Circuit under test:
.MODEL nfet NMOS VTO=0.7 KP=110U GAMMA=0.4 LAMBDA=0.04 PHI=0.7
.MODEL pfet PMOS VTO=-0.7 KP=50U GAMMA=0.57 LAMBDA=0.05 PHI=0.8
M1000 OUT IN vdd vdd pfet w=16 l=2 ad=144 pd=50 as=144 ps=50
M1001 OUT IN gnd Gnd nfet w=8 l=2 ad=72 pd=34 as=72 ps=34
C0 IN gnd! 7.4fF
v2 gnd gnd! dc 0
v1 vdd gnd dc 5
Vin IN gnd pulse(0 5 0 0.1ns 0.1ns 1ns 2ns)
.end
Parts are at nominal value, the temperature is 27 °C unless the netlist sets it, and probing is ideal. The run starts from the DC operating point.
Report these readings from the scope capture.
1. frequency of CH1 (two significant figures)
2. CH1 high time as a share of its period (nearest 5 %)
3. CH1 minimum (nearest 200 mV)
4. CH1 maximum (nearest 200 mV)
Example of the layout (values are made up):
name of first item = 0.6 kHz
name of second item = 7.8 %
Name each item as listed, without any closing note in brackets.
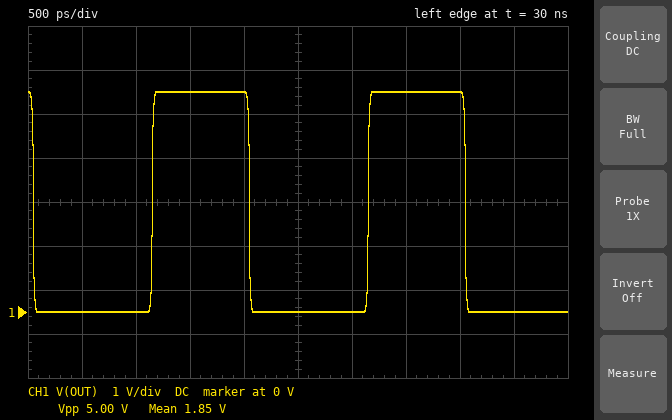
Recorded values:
frequency of CH1 = 500 MHz
CH1 high time as a share of its period = 45 %
CH1 minimum = 0 V
CH1 maximum = 5.0 V
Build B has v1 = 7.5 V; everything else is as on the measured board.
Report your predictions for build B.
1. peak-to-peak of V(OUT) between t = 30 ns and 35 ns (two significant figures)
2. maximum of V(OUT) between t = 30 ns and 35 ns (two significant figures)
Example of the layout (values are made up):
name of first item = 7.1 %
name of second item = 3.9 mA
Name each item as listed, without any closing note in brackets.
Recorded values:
peak-to-peak of V(OUT) between t = 30 ns and 35 ns = 7.0 V
maximum of V(OUT) between t = 30 ns and 35 ns = 7.5 V
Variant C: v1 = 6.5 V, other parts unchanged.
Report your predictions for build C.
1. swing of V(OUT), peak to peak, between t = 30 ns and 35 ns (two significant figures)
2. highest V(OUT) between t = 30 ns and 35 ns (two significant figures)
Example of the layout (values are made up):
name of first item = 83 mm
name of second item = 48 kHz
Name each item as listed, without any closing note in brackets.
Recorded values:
swing of V(OUT), peak to peak, between t = 30 ns and 35 ns = 6.4 V
highest V(OUT) between t = 30 ns and 35 ns = 6.5 V
